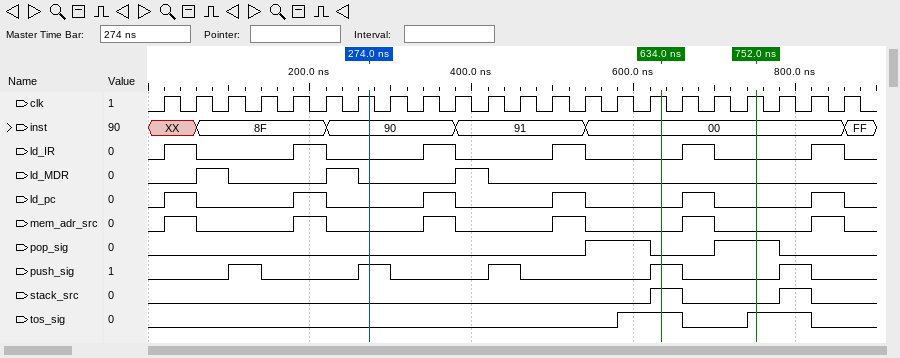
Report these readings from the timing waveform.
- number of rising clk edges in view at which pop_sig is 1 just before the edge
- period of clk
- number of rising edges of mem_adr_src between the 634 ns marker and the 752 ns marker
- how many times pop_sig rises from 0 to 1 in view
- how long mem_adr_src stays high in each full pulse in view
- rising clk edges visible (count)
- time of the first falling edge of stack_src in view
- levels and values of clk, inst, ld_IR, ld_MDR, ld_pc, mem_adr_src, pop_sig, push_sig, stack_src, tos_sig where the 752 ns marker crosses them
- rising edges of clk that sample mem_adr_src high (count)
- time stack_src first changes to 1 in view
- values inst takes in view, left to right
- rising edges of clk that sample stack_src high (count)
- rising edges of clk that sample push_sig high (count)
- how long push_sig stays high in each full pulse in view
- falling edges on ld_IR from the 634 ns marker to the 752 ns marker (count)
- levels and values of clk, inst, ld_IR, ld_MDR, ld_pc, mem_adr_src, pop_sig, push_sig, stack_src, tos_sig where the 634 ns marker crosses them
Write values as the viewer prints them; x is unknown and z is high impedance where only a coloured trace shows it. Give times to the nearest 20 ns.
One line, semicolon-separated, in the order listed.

4; 40 ns; 1; 2; 40 ns, 40 ns, 40 ns, 40 ns, 40 ns, 40 ns; 22; 660 ns; clk=1, inst=00, ld_IR=0, ld_MDR=0, ld_pc=0, mem_adr_src=0, pop_sig=1, push_sig=0, stack_src=0, tos_sig=1; 6; 620 ns; XX, 8F, 90, 91, 00, FF; 2; 5; 40 ns, 40 ns, 40 ns, 40 ns, 40 ns; 1; clk=1, inst=00, ld_IR=0, ld_MDR=0, ld_pc=0, mem_adr_src=0, pop_sig=0, push_sig=1, stack_src=1, tos_sig=1
